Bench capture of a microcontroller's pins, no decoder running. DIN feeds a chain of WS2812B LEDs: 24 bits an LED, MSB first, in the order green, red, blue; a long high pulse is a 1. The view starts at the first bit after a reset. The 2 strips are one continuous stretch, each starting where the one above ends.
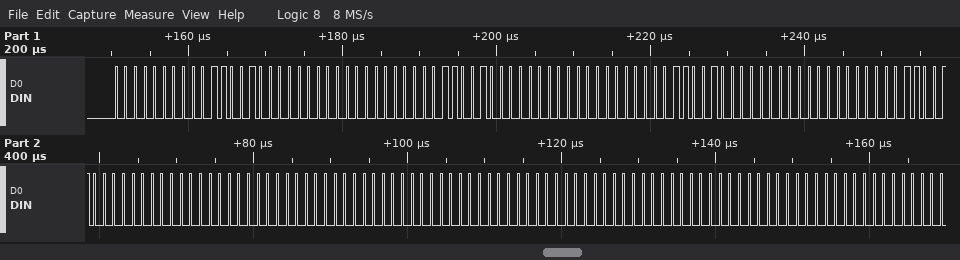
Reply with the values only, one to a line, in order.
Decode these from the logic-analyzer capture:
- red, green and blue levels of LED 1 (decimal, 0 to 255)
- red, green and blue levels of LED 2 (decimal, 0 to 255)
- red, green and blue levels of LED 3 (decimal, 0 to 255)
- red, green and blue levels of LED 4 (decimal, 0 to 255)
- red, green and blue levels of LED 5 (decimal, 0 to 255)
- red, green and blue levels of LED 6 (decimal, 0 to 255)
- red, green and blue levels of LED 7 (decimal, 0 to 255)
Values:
50, 0, 0
50, 0, 0
50, 0, 0
50, 0, 0
0, 0, 0
0, 0, 0
0, 0, 0
